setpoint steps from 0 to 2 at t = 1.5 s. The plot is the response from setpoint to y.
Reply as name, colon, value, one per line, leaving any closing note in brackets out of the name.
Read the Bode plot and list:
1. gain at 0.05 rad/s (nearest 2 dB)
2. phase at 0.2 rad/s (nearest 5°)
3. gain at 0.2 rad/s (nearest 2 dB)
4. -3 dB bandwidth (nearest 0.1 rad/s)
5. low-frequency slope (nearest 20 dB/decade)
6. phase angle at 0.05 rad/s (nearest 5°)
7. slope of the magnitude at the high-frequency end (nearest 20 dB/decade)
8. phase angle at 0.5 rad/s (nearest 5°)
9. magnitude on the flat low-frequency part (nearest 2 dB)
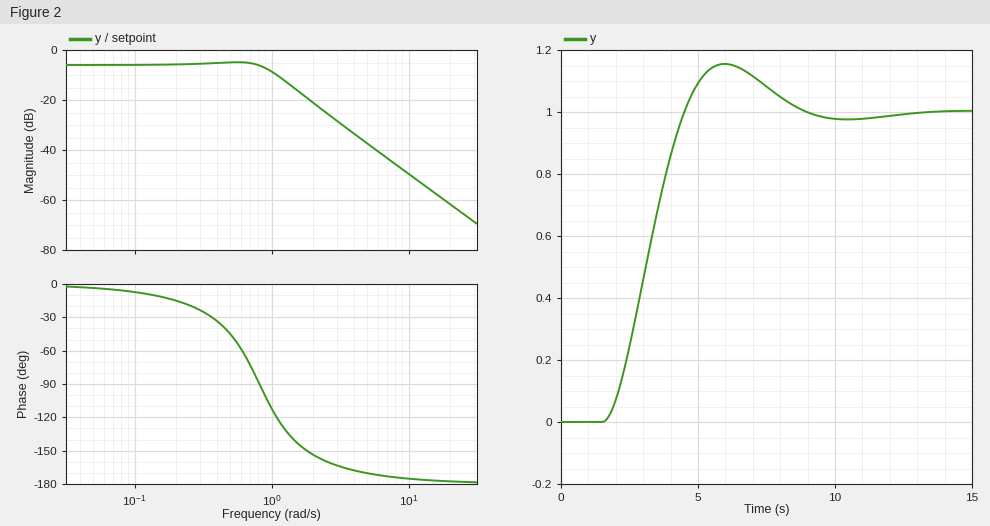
gain at 0.05 rad/s: -6 dB
phase at 0.2 rad/s: -15°
gain at 0.2 rad/s: -6 dB
-3 dB bandwidth: 1.0 rad/s
low-frequency slope: 0 dB/decade
phase angle at 0.05 rad/s: -5°
slope of the magnitude at the high-frequency end: -40 dB/decade
phase angle at 0.5 rad/s: -45°
magnitude on the flat low-frequency part: -6 dB
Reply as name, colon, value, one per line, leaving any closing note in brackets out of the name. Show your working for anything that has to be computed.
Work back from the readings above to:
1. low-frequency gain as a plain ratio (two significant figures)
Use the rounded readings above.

low-frequency gain as a plain ratio: 10^(-6 / 20) = 0.50
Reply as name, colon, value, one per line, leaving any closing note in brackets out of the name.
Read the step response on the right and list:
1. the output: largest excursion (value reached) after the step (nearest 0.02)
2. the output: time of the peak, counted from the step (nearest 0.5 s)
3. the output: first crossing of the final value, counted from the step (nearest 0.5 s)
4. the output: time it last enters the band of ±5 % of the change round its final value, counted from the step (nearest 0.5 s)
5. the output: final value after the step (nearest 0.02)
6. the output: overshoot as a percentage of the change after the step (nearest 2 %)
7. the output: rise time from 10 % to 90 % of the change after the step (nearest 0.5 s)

the output: largest excursion (value reached) after the step: 1.16
the output: time of the peak, counted from the step: 4.5 s
the output: first crossing of the final value, counted from the step: 3.0 s
the output: time it last enters the band of ±5 % of the change round its final value, counted from the step: 6.5 s
the output: final value after the step: 1.00
the output: overshoot as a percentage of the change after the step: 16 %
the output: rise time from 10 % to 90 % of the change after the step: 2.0 s
